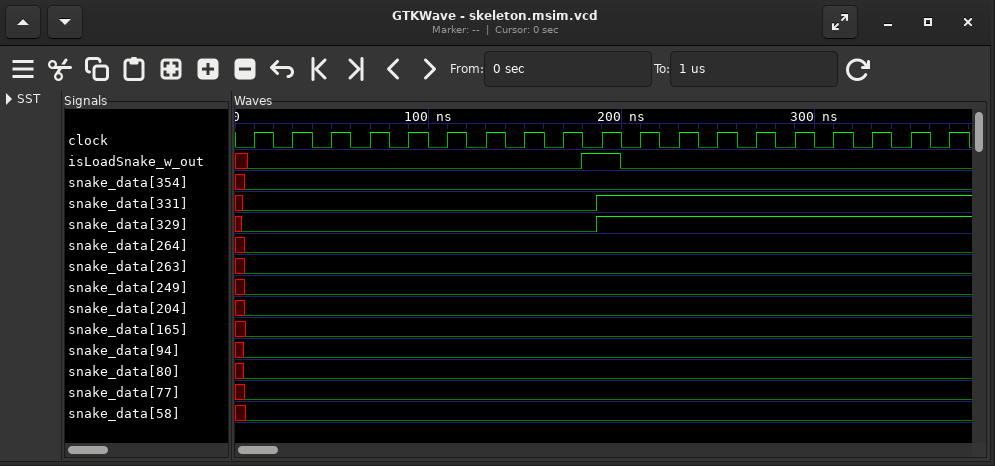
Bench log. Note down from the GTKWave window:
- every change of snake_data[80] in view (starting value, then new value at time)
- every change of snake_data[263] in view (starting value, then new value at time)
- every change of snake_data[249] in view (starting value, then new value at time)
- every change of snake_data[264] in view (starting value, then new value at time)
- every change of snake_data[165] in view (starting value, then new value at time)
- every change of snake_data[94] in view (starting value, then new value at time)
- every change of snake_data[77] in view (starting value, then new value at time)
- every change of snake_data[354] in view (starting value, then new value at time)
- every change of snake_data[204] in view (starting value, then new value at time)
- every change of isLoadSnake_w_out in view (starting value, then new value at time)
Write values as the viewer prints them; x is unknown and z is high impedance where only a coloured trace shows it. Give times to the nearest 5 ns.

x, 0 at 5 ns
x, 0 at 5 ns
x, 0 at 5 ns
x, 0 at 5 ns
x, 0 at 5 ns
x, 0 at 5 ns
x, 0 at 5 ns
x, 0 at 5 ns
x, 0 at 5 ns
x, 0 at 5 ns, 1 at 180 ns, 0 at 200 ns
